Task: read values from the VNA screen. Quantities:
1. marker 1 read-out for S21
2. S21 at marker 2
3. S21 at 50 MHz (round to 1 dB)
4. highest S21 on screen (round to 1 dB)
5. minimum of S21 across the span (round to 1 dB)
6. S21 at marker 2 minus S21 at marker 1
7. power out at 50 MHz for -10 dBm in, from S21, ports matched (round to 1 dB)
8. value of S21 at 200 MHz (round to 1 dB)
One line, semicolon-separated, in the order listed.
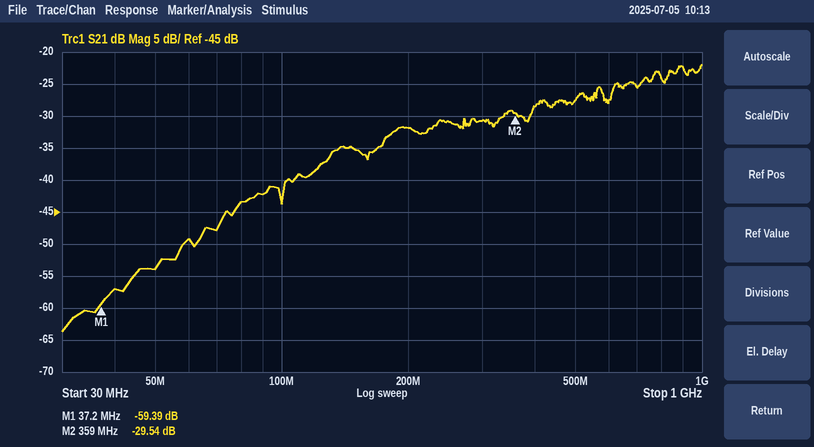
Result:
-59.39 dB; -29.54 dB; -54 dB; -22 dB; -64 dB; 29.85 dB; -64 dBm; -32 dB
